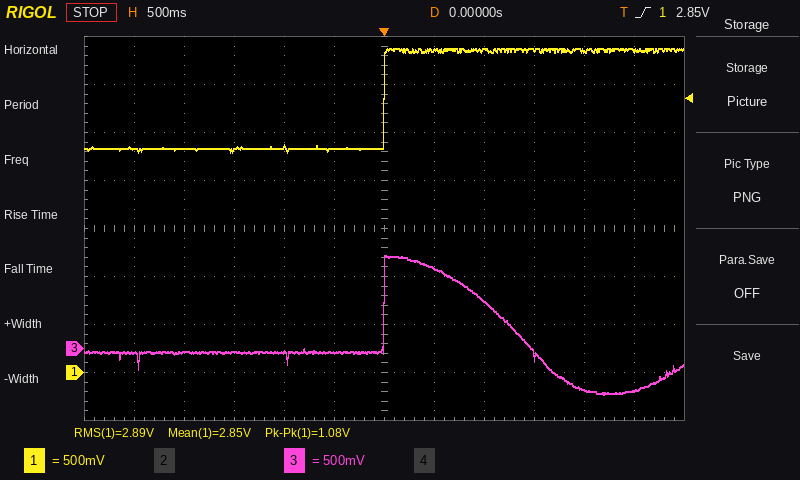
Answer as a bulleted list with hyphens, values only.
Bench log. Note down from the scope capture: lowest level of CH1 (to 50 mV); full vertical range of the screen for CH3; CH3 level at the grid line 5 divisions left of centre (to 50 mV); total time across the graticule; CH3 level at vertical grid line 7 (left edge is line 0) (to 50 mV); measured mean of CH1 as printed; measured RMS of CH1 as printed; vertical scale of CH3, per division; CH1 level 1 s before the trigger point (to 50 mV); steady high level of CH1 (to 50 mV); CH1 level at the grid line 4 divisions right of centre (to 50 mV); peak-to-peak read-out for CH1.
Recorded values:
- 2.30 V
- 4 V
- -50 mV
- 6 s
- 850 mV
- 2.85 V
- 2.89 V
- 500 mV
- 2.35 V
- 3.35 V
- 3.35 V
- 1.08 V
